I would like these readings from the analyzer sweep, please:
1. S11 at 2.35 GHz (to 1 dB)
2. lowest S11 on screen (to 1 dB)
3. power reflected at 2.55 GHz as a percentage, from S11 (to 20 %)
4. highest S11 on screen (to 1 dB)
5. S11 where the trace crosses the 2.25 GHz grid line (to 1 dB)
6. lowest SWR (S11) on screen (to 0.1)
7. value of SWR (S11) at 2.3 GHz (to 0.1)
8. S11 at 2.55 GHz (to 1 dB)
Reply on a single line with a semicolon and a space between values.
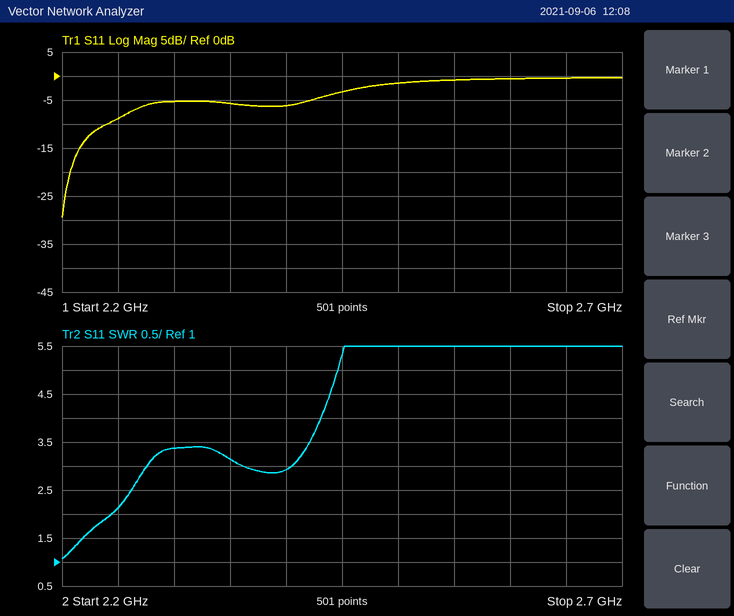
-6 dB; -29 dB; 80 %; 0 dB; -9 dB; 1.1; 3.4; -1 dB
